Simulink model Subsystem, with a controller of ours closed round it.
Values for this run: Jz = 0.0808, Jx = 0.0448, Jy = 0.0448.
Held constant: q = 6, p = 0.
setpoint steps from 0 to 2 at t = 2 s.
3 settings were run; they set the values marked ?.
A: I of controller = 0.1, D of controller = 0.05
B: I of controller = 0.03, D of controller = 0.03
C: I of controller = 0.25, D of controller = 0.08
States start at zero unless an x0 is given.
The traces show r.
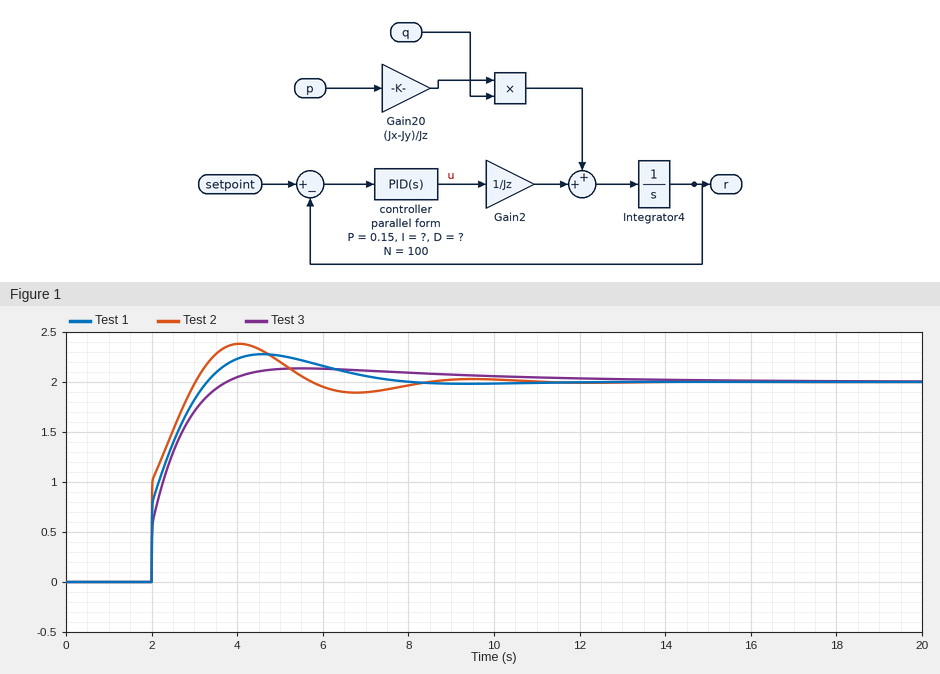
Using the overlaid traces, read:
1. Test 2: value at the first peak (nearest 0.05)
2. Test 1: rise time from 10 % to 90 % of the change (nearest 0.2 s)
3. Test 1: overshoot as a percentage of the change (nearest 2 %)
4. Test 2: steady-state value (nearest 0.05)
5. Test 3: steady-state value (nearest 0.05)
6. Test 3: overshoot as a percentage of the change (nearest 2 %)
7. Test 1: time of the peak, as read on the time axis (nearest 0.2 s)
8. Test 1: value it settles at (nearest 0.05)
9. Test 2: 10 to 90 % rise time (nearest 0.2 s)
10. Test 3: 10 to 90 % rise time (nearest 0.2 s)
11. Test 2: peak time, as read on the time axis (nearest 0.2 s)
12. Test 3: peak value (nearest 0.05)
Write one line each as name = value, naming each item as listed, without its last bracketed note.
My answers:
Test 2: value at the first peak = 2.40
Test 1: rise time from 10 % to 90 % of the change = 1.0 s
Test 1: overshoot as a percentage of the change = 14 %
Test 2: steady-state value = 2.00
Test 3: steady-state value = 2.00
Test 3: overshoot as a percentage of the change = 6 %
Test 1: time of the peak, as read on the time axis = 4.6 s
Test 1: value it settles at = 2.00
Test 2: 10 to 90 % rise time = 0.8 s
Test 3: 10 to 90 % rise time = 1.2 s
Test 2: peak time, as read on the time axis = 4.0 s
Test 3: peak value = 2.15
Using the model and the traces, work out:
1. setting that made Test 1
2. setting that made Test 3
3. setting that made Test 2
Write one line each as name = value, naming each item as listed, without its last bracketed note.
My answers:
setting that made Test 1 = A
setting that made Test 3 = B
setting that made Test 2 = C
